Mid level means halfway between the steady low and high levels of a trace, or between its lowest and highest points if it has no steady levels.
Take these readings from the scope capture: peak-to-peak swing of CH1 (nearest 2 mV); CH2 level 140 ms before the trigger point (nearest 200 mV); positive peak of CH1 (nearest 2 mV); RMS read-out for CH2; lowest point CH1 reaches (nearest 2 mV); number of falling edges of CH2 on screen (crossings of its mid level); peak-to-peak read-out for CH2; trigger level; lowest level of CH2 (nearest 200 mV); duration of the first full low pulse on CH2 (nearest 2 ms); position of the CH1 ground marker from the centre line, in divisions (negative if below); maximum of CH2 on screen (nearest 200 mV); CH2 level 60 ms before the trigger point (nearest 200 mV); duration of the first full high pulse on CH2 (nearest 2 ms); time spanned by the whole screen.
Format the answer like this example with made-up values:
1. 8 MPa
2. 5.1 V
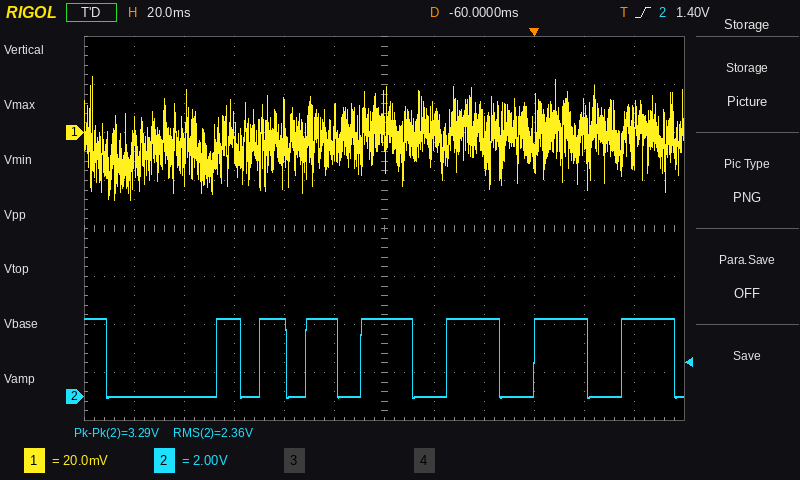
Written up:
1. 52 mV
2. 0.0 V
3. 24 mV
4. 2.36 V
5. -28 mV
6. 8
7. 3.29 V
8. 1.40 V
9. 0.0 V
10. 44 ms
11. +2.0 div
12. 3.2 V
13. 3.2 V
14. 10 ms
15. 240 ms
